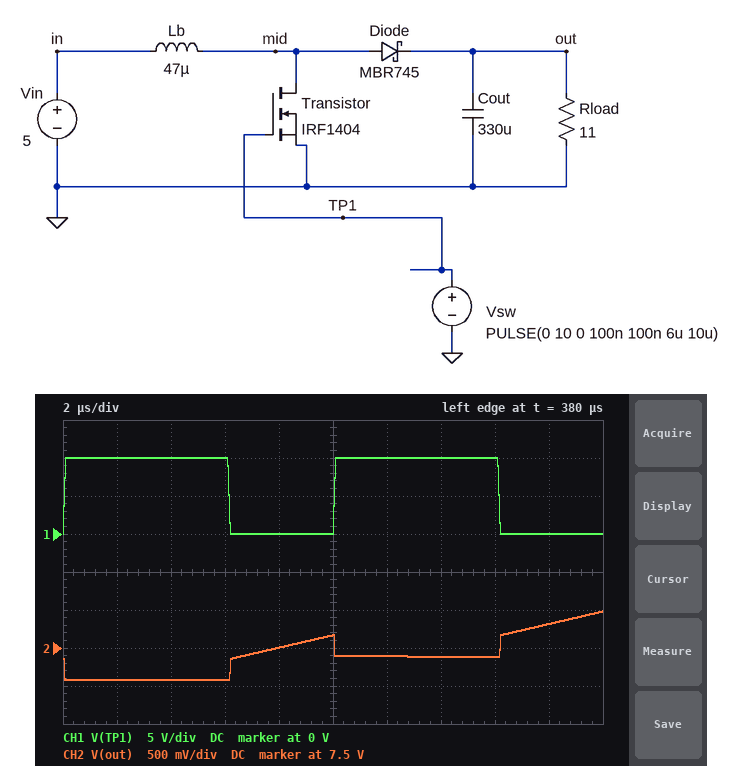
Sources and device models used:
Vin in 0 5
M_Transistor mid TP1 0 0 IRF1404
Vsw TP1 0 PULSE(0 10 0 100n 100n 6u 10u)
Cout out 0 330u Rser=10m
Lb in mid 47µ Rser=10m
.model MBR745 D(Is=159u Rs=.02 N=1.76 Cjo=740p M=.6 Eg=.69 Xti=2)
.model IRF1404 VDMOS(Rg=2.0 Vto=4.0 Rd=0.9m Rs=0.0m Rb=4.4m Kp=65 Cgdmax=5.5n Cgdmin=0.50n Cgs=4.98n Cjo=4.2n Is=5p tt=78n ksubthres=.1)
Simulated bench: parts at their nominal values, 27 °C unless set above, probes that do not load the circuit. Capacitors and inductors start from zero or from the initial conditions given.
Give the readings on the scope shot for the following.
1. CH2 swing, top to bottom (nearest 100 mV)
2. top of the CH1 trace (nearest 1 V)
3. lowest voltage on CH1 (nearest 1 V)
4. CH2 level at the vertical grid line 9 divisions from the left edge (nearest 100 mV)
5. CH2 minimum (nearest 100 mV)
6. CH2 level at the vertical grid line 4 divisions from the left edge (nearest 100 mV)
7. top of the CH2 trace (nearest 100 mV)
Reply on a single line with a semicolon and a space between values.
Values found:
900 mV; 10 V; 0 V; 7.8 V; 7.1 V; 7.5 V; 8.0 V
